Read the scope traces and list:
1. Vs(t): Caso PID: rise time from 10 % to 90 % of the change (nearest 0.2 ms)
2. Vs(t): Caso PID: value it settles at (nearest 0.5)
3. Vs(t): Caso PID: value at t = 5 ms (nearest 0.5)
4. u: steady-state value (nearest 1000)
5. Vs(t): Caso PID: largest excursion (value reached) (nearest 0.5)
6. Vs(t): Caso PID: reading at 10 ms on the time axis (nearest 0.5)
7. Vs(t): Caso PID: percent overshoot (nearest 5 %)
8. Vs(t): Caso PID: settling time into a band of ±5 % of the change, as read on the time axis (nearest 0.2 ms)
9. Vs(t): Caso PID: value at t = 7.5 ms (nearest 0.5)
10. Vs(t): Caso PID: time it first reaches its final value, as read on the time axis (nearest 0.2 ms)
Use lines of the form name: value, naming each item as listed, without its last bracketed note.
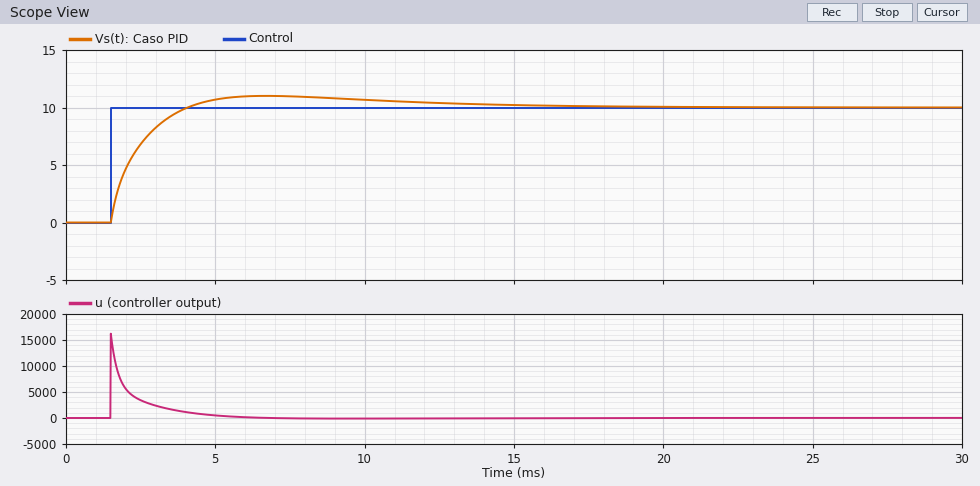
Vs(t): Caso PID: rise time from 10 % to 90 % of the change: 1.8 ms
Vs(t): Caso PID: value it settles at: 10.0
Vs(t): Caso PID: value at t = 5 ms: 10.5
u: steady-state value: 0
Vs(t): Caso PID: largest excursion (value reached): 11.0
Vs(t): Caso PID: reading at 10 ms on the time axis: 10.5
Vs(t): Caso PID: percent overshoot: 10 %
Vs(t): Caso PID: settling time into a band of ±5 % of the change, as read on the time axis: 11.4 ms
Vs(t): Caso PID: value at t = 7.5 ms: 11.0
Vs(t): Caso PID: time it first reaches its final value, as read on the time axis: 4.0 ms
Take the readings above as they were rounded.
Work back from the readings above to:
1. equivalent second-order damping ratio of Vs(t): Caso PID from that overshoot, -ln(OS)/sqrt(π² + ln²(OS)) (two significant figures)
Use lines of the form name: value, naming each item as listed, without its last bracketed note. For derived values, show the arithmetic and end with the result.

equivalent second-order damping ratio of Vs(t): Caso PID from that overshoot, -ln(OS)/sqrt(π² + ln²(OS)): ln(0.1) = -2.303; 2.303 / sqrt(9.870 + 5.302) = 0.59
